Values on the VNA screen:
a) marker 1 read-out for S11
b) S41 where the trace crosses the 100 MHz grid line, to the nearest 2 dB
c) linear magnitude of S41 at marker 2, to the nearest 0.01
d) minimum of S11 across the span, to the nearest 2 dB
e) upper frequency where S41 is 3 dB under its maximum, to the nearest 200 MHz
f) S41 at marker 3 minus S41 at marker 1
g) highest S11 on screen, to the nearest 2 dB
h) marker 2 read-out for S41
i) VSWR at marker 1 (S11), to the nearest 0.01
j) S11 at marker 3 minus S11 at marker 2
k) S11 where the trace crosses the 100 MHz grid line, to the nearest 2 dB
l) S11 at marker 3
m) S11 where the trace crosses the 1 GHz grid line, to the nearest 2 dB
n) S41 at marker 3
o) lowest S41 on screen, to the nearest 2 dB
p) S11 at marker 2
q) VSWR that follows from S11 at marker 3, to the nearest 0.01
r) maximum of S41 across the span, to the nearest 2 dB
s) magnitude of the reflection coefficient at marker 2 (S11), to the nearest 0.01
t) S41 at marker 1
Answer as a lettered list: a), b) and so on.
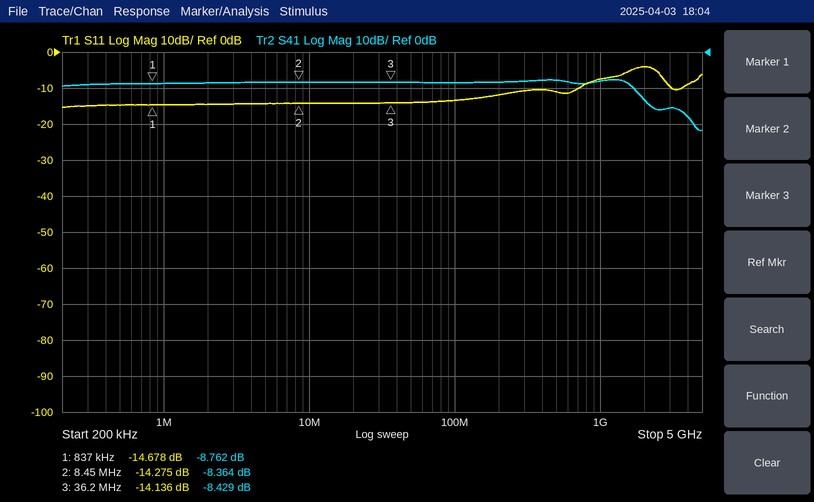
a) -14.678 dB
b) -8 dB
c) 0.38
d) -16 dB
e) 1.8 GHz
f) 0.333 dB
g) -4 dB
h) -8.364 dB
i) 1.45
j) 0.139 dB
k) -14 dB
l) -14.136 dB
m) -8 dB
n) -8.429 dB
o) -22 dB
p) -14.275 dB
q) 1.49
r) -8 dB
s) 0.19
t) -8.762 dB
